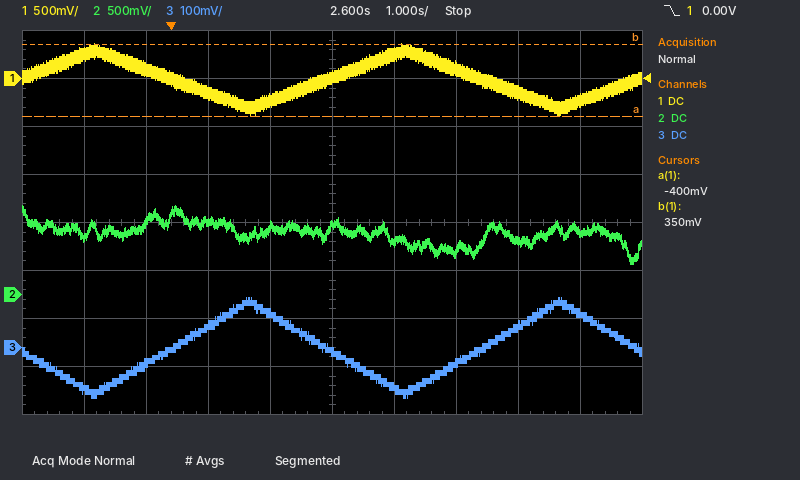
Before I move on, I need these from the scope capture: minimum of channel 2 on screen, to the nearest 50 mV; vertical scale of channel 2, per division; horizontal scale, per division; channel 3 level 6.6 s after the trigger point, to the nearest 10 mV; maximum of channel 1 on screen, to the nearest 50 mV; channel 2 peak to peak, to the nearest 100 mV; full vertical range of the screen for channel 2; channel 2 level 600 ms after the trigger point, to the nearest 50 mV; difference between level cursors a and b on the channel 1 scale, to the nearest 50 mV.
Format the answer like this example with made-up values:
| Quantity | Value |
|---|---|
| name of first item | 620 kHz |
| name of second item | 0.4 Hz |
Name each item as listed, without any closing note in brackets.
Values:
| Quantity | Value |
|---|---|
| minimum of channel 2 on screen, to the nearest 50 mV | 300 mV |
| vertical scale of channel 2, per division | 500 mV |
| horizontal scale, per division | 1 s |
| channel 3 level 6.6 s after the trigger point, to the nearest 10 mV | 70 mV |
| maximum of channel 1 on screen, to the nearest 50 mV | 350 mV |
| channel 2 peak to peak, to the nearest 100 mV | 600 mV |
| full vertical range of the screen for channel 2 | 4 V |
| channel 2 level 600 ms after the trigger point, to the nearest 50 mV | 750 mV |
| difference between level cursors a and b on the channel 1 scale, to the nearest 50 mV | 750 mV |
